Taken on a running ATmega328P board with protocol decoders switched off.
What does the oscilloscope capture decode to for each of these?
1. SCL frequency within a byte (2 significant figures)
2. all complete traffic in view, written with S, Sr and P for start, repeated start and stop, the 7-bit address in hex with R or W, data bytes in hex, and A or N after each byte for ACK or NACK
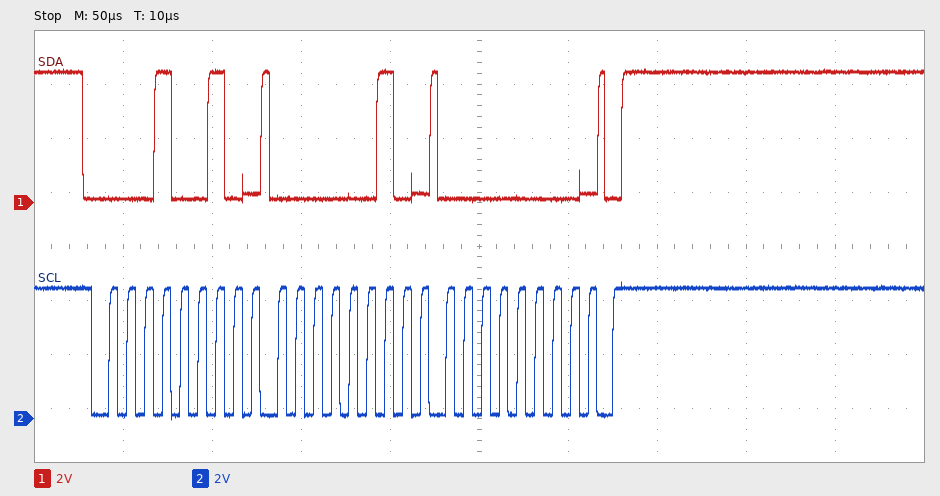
100 kHz
S 09W A 02 A 00 A P
